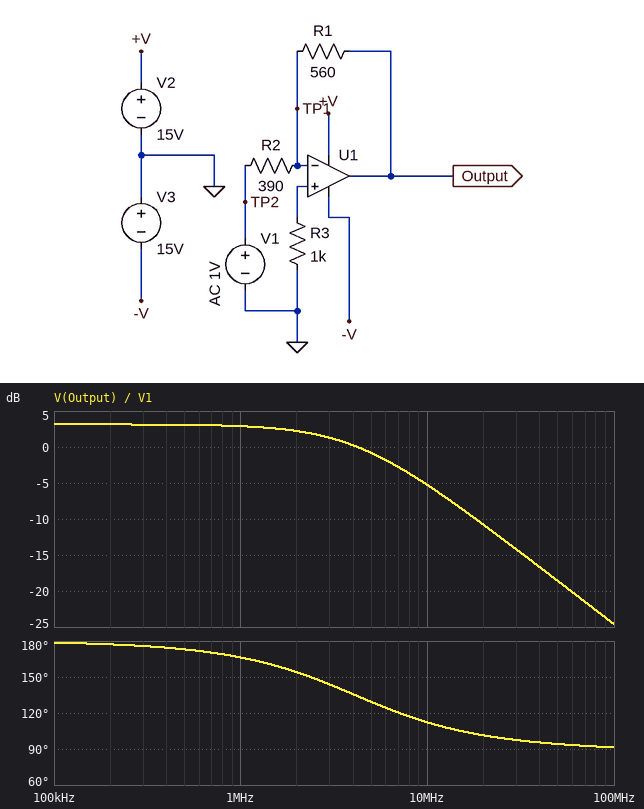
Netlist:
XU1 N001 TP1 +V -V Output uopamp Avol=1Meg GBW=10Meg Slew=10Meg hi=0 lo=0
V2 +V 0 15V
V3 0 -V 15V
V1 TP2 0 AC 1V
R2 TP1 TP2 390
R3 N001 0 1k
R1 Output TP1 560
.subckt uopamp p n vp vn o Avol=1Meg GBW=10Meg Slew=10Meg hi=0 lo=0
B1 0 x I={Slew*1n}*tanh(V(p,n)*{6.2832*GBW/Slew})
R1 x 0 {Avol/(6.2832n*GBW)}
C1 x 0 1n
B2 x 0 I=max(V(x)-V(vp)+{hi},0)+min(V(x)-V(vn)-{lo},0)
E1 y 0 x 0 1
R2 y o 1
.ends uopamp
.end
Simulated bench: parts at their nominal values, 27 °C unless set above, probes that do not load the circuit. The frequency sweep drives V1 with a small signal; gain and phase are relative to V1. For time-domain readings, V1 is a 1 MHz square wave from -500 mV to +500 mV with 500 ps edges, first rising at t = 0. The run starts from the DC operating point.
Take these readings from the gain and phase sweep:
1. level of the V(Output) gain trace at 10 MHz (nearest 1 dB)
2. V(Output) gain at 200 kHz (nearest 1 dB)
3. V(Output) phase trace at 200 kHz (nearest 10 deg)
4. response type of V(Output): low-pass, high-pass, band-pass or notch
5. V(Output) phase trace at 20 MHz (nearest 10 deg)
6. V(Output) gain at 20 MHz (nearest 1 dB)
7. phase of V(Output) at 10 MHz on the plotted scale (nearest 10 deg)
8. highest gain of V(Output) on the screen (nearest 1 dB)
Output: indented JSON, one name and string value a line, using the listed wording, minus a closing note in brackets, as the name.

{
  "level of the V(Output) gain trace at 10 MHz": "-5 dB",
  "V(Output) gain at 200 kHz": "3 dB",
  "V(Output) phase trace at 200 kHz": "180 deg",
  "response type of V(Output): low-pass, high-pass, band-pass or notch": "low-pass",
  "V(Output) phase trace at 20 MHz": "100 deg",
  "V(Output) gain at 20 MHz": "-11 dB",
  "phase of V(Output) at 10 MHz on the plotted scale": "110 deg",
  "highest gain of V(Output) on the screen": "3 dB"
}
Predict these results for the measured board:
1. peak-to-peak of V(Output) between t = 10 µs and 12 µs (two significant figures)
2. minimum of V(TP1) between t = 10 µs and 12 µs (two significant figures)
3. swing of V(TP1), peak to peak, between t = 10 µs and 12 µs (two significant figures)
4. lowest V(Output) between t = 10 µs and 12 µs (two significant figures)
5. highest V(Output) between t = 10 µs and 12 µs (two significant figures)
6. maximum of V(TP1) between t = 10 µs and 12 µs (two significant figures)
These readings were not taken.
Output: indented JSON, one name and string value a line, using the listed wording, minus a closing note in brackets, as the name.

{
  "peak-to-peak of V(Output) between t = 10 µs and 12 µs": "1.4 V",
  "minimum of V(TP1) between t = 10 µs and 12 µs": "-590 mV",
  "swing of V(TP1), peak to peak, between t = 10 µs and 12 µs": "1.2 V",
  "lowest V(Output) between t = 10 µs and 12 µs": "-720 mV",
  "highest V(Output) between t = 10 µs and 12 µs": "720 mV",
  "maximum of V(TP1) between t = 10 µs and 12 µs": "590 mV"
}
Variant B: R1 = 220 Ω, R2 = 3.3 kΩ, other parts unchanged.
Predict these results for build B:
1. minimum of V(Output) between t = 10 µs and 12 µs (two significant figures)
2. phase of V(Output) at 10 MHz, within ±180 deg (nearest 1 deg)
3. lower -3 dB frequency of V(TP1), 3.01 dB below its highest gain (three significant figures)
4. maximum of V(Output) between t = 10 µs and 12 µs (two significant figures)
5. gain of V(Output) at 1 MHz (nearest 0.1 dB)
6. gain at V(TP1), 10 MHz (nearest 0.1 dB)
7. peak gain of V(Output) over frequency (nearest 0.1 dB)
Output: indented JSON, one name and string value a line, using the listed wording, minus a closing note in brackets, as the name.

{
  "minimum of V(Output) between t = 10 µs and 12 µs": "-33 mV",
  "phase of V(Output) at 10 MHz, within ±180 deg": "133 deg",
  "lower -3 dB frequency of V(TP1), 3.01 dB below its highest gain": "9.37 MHz",
  "maximum of V(Output) between t = 10 µs and 12 µs": "33 mV",
  "gain of V(Output) at 1 MHz": "-23.6 dB",
  "gain at V(TP1), 10 MHz": "-26.8 dB",
  "peak gain of V(Output) over frequency": "-23.5 dB"
}
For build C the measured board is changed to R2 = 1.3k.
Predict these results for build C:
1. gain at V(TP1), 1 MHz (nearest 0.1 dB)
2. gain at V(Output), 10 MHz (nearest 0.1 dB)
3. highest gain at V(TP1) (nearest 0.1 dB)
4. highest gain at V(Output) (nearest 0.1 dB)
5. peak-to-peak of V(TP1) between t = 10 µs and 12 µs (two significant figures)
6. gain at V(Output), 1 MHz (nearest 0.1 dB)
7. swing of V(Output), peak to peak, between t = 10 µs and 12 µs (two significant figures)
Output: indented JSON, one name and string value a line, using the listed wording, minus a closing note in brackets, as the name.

{
  "gain at V(TP1), 1 MHz": "-27.4 dB",
  "gain at V(Output), 10 MHz": "-12.2 dB",
  "highest gain at V(TP1)": "-10.4 dB",
  "highest gain at V(Output)": "-7.3 dB",
  "peak-to-peak of V(TP1) between t = 10 µs and 12 µs": "600 mV",
  "gain at V(Output), 1 MHz": "-7.4 dB",
  "swing of V(Output), peak to peak, between t = 10 µs and 12 µs": "430 mV"
}
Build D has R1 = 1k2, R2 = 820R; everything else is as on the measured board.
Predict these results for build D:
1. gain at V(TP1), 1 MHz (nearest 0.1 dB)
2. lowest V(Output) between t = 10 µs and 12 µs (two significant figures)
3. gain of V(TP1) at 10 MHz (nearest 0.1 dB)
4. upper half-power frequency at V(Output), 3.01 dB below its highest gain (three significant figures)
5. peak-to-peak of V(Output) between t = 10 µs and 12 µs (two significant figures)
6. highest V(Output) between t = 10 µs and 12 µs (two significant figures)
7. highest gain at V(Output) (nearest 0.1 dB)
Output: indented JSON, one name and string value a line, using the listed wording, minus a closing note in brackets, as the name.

{
  "gain at V(TP1), 1 MHz": "-16.9 dB",
  "lowest V(Output) between t = 10 µs and 12 µs": "-730 mV",
  "gain of V(TP1) at 10 MHz": "-5.2 dB",
  "upper half-power frequency at V(Output), 3.01 dB below its highest gain": "4.06 MHz",
  "peak-to-peak of V(Output) between t = 10 µs and 12 µs": "1.5 V",
  "highest V(Output) between t = 10 µs and 12 µs": "730 mV",
  "highest gain at V(Output)": "3.3 dB"
}
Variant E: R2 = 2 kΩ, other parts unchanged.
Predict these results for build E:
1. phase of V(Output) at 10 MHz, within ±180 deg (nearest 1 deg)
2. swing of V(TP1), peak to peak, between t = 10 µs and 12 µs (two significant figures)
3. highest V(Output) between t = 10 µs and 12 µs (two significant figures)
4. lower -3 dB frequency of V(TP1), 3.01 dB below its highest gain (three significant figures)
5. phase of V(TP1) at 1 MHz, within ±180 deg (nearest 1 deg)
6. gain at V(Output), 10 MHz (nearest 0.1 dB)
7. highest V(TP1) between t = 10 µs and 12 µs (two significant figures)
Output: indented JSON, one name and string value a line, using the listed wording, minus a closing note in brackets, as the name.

{
  "phase of V(Output) at 10 MHz, within ±180 deg": "128 deg",
  "swing of V(TP1), peak to peak, between t = 10 µs and 12 µs": "430 mV",
  "highest V(Output) between t = 10 µs and 12 µs": "140 mV",
  "lower -3 dB frequency of V(TP1), 3.01 dB below its highest gain": "7.81 MHz",
  "phase of V(TP1) at 1 MHz, within ±180 deg": "83 deg",
  "gain at V(Output), 10 MHz": "-15.3 dB",
  "highest V(TP1) between t = 10 µs and 12 µs": "220 mV"
}
